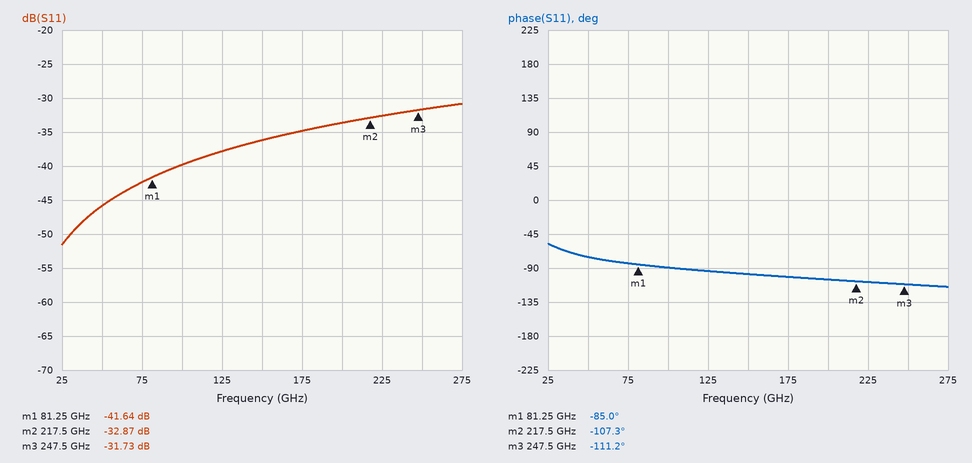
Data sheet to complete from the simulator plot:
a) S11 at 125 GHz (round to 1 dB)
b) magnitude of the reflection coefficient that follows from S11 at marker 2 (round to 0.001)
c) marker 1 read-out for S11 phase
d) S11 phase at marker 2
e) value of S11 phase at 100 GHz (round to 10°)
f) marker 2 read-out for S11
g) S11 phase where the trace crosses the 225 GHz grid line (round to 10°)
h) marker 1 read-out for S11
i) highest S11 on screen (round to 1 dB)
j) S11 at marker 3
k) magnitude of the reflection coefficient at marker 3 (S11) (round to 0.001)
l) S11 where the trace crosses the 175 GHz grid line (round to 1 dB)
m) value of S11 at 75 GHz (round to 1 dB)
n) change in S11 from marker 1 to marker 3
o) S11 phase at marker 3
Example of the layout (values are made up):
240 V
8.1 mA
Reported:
-38 dB
0.023
-85.0°
-107.3°
-90°
-32.87 dB
-110°
-41.64 dB
-31 dB
-31.73 dB
0.026
-35 dB
-42 dB
9.91 dB
-111.2°
